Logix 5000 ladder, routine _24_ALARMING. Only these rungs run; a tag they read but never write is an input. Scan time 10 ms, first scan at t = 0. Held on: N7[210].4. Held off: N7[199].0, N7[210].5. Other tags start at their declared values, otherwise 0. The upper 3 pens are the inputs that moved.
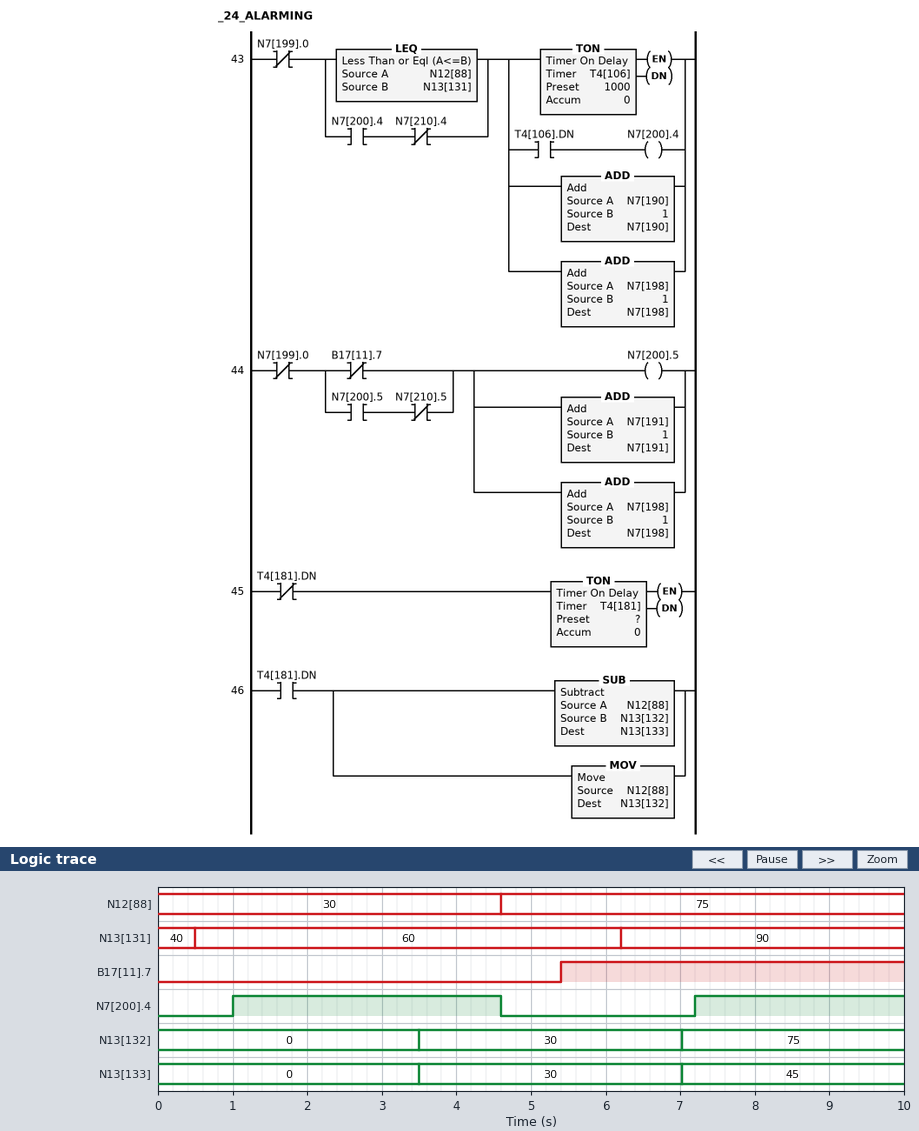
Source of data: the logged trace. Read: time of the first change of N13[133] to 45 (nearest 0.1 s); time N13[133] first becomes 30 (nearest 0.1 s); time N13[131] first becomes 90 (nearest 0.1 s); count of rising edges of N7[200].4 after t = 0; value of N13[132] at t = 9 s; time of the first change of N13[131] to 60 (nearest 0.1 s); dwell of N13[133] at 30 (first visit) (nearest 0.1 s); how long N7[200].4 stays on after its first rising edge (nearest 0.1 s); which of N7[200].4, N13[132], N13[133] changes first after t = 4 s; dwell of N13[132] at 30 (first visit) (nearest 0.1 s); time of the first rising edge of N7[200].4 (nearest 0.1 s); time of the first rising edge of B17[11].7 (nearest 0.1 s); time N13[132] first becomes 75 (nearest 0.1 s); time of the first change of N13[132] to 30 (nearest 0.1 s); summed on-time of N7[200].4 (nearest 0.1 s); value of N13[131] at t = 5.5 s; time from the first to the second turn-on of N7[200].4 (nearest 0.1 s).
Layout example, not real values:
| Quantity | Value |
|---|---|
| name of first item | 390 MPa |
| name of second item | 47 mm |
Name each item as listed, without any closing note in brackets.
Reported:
| Quantity | Value |
|---|---|
| time of the first change of N13[133] to 45 | 7.0 s |
| time N13[133] first becomes 30 | 3.5 s |
| time N13[131] first becomes 90 | 6.2 s |
| count of rising edges of N7[200].4 after t = 0 | 2 |
| value of N13[132] at t = 9 s | 75 |
| time of the first change of N13[131] to 60 | 0.5 s |
| dwell of N13[133] at 30 (first visit) | 3.5 s |
| how long N7[200].4 stays on after its first rising edge | 3.6 s |
| which of N7[200].4, N13[132], N13[133] changes first after t = 4 s | N7[200].4 |
| dwell of N13[132] at 30 (first visit) | 3.5 s |
| time of the first rising edge of N7[200].4 | 1.0 s |
| time of the first rising edge of B17[11].7 | 5.4 s |
| time N13[132] first becomes 75 | 7.0 s |
| time of the first change of N13[132] to 30 | 3.5 s |
| summed on-time of N7[200].4 | 6.4 s |
| value of N13[131] at t = 5.5 s | 60 |
| time from the first to the second turn-on of N7[200].4 | 6.2 s |
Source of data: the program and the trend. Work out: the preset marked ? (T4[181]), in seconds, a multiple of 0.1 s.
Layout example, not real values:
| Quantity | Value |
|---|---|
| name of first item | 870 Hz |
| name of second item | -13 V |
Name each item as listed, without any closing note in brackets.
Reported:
| Quantity | Value |
|---|---|
| the preset marked ? (T4[181]), in seconds, a multiple of 0.1 s | 3.5 s |
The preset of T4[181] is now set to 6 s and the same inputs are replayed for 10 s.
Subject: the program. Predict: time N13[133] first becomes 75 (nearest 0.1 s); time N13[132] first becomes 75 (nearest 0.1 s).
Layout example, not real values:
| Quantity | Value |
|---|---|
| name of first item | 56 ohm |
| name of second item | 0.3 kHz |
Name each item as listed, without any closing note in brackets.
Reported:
| Quantity | Value |
|---|---|
| time N13[133] first becomes 75 | 6.0 s |
| time N13[132] first becomes 75 | 6.0 s |
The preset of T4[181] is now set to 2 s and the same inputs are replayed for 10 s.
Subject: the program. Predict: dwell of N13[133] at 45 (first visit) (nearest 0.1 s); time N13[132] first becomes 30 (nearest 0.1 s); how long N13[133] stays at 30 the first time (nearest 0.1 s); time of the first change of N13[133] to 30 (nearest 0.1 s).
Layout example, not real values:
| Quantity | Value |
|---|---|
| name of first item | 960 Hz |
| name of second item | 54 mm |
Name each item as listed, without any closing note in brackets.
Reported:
| Quantity | Value |
|---|---|
| dwell of N13[133] at 45 (first visit) | 2.0 s |
| time N13[132] first becomes 30 | 2.0 s |
| how long N13[133] stays at 30 the first time | 2.0 s |
| time of the first change of N13[133] to 30 | 2.0 s |
